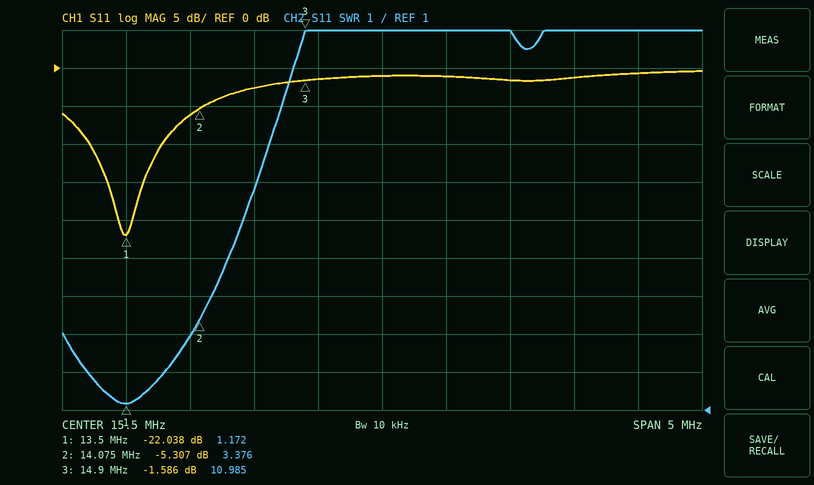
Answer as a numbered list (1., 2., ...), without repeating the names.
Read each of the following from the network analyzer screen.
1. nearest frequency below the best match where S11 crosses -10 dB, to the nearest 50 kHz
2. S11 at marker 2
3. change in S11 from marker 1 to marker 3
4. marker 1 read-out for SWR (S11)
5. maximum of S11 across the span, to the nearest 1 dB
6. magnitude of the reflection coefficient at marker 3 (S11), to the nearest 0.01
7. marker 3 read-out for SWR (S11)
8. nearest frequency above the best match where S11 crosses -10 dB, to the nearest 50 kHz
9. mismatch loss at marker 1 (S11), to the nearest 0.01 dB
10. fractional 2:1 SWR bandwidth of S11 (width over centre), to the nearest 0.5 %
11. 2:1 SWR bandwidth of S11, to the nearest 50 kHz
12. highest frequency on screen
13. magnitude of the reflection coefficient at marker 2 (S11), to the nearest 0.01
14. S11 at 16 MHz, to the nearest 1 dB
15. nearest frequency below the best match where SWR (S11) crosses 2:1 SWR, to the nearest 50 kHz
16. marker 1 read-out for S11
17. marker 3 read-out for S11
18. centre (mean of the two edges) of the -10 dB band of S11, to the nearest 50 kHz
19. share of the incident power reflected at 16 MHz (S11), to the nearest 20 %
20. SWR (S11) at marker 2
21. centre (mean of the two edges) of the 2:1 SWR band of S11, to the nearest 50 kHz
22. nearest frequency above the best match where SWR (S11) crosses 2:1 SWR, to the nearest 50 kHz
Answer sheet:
1. 13.20 MHz
2. -5.307 dB
3. 20.452 dB
4. 1.172
5. 0 dB
6. 0.83
7. 10.985
8. 13.80 MHz
9. 0.03 dB
10. 4.5 %
11. 600 kHz
12. 18 MHz
13. 0.54
14. -1 dB
15. 13.20 MHz
16. -22.038 dB
17. -1.586 dB
18. 13.50 MHz
19. 80 %
20. 3.376
21. 13.50 MHz
22. 13.80 MHz
